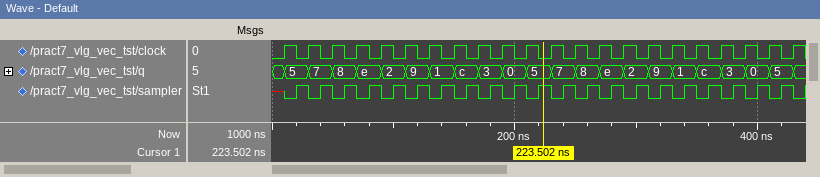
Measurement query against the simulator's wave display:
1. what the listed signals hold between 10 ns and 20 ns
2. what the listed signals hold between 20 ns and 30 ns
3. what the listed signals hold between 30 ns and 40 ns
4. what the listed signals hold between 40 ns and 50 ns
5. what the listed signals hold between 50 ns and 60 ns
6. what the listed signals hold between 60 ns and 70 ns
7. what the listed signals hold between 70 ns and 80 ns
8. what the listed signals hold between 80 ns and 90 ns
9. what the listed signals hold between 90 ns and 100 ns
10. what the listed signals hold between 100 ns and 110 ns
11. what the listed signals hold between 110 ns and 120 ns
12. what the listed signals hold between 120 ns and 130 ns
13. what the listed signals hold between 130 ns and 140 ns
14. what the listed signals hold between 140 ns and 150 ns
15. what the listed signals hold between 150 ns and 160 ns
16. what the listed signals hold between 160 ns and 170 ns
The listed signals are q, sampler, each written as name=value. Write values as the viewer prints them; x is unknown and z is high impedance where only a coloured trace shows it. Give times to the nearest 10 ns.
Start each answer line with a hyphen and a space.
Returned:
- q=5, sampler=0
- q=5, sampler=1
- q=7, sampler=0
- q=7, sampler=1
- q=8, sampler=0
- q=8, sampler=1
- q=e, sampler=0
- q=e, sampler=1
- q=2, sampler=0
- q=2, sampler=1
- q=9, sampler=0
- q=9, sampler=1
- q=1, sampler=0
- q=1, sampler=1
- q=c, sampler=0
- q=c, sampler=1
